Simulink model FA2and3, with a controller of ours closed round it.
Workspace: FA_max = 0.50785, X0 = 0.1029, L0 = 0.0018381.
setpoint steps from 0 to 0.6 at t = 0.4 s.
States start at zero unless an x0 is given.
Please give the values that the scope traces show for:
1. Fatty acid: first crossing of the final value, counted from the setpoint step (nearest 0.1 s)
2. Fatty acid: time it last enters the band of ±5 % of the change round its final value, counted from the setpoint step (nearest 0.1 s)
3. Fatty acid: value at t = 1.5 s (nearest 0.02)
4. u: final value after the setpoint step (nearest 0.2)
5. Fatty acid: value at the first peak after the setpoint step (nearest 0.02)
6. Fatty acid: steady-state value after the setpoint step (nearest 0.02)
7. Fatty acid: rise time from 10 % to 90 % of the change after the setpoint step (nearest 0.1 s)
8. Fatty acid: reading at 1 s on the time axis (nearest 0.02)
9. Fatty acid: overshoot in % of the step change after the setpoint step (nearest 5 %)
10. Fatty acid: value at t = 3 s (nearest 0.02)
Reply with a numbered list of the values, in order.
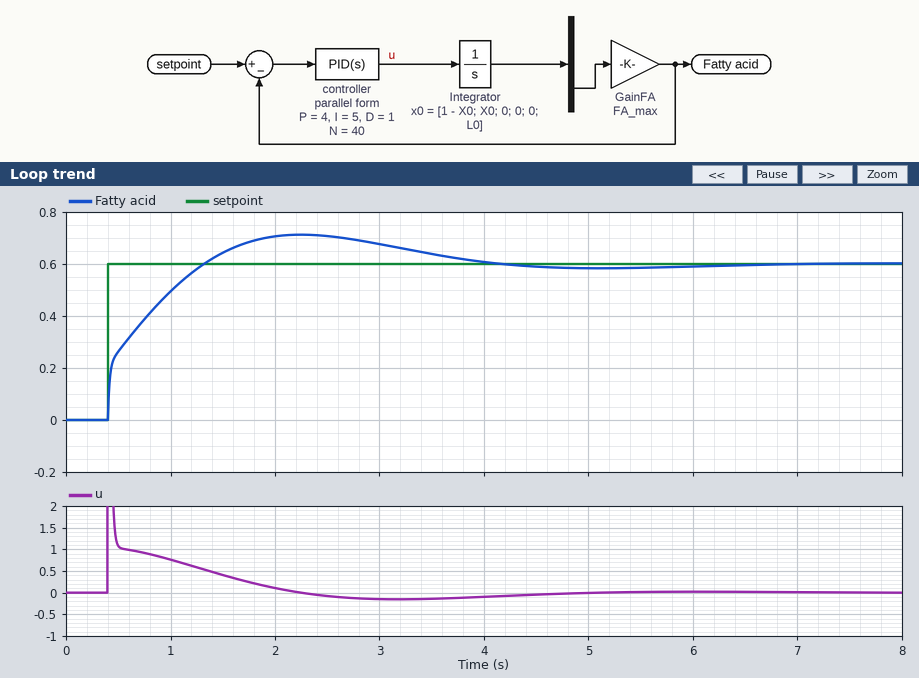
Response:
1. 0.9 s
2. 3.2 s
3. 0.64
4. 0.0
5. 0.72
6. 0.60
7. 0.7 s
8. 0.50
9. 20 %
10. 0.68
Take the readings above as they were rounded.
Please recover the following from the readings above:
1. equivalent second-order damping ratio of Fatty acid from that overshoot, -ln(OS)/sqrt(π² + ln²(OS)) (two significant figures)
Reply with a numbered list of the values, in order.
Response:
1. 0.46
